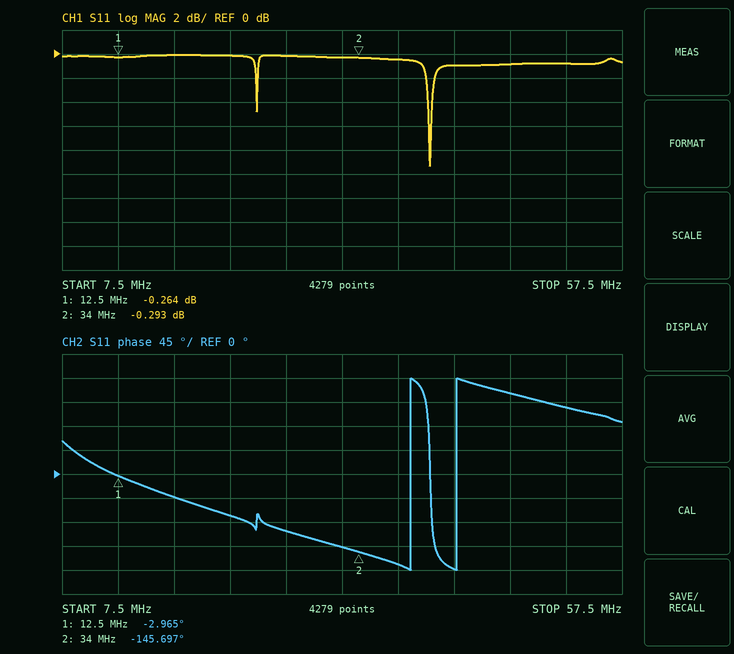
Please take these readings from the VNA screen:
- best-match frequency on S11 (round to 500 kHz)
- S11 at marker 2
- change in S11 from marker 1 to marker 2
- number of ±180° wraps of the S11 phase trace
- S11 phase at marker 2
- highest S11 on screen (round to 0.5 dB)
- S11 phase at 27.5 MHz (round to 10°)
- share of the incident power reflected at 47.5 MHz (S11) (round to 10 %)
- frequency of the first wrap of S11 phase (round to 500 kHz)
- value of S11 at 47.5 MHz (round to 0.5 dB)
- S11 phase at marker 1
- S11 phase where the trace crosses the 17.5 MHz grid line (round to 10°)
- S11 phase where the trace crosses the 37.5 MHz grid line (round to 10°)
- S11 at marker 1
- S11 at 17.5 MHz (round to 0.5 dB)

40.5 MHz
-0.293 dB
-0.029 dB
2
-145.697°
0.0 dB
-110°
80 %
38.5 MHz
-1.0 dB
-2.965°
-40°
-170°
-0.264 dB
0.0 dB
